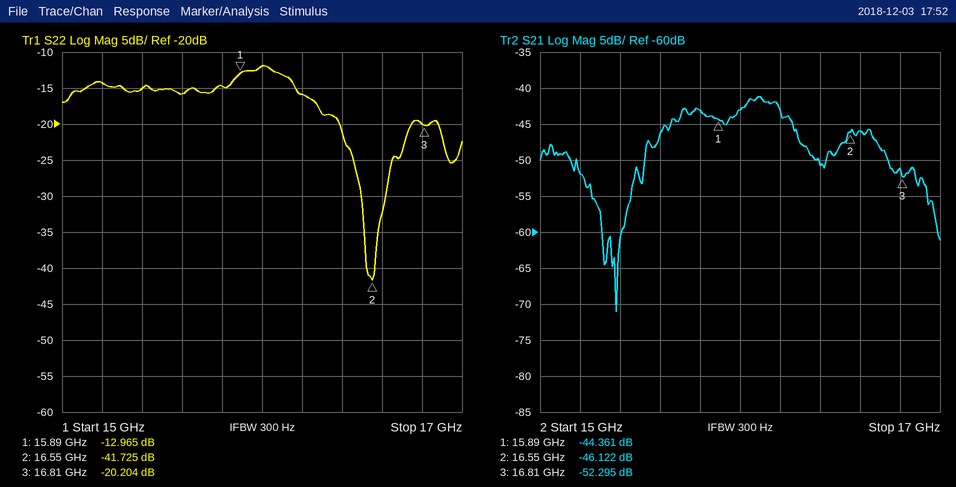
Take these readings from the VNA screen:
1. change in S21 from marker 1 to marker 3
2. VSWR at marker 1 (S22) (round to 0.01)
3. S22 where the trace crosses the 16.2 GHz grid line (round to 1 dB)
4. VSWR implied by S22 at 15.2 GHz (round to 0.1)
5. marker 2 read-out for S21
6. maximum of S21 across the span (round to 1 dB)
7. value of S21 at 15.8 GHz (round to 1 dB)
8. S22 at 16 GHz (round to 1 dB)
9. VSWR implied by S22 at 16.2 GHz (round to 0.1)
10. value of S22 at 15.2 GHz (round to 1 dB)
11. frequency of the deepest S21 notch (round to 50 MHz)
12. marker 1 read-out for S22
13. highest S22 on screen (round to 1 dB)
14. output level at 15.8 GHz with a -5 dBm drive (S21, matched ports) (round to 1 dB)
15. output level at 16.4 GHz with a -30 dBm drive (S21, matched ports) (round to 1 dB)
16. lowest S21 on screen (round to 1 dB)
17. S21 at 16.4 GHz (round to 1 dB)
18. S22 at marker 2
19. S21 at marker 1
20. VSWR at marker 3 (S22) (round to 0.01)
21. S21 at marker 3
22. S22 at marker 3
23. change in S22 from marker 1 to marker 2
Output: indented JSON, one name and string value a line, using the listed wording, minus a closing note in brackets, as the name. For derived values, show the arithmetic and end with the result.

{
  "change in S21 from marker 1 to marker 3": "-52.295 − (-44.361) = -7.934 dB",
  "VSWR at marker 1 (S22)": "(1 + 0.2248)/(1 − 0.2248) ≈ 1.58",
  "S22 where the trace crosses the 16.2 GHz grid line": "-16 dB",
  "VSWR implied by S22 at 15.2 GHz": "|Γ| = 10^(-14/20) = 0.1995; VSWR = (1 + 0.1995)/(1 − 0.1995) ≈ 1.5",
  "marker 2 read-out for S21": "-46.122 dB",
  "maximum of S21 across the span": "-41 dB",
  "value of S21 at 15.8 GHz": "-43 dB",
  "S22 at 16 GHz": "-12 dB",
  "VSWR implied by S22 at 16.2 GHz": "|Γ| = 10^(-16/20) = 0.1585; VSWR = (1 + 0.1585)/(1 − 0.1585) ≈ 1.4",
  "value of S22 at 15.2 GHz": "-14 dB",
  "frequency of the deepest S21 notch": "15.40 GHz",
  "marker 1 read-out for S22": "-12.965 dB",
  "highest S22 on screen": "-12 dB",
  "output level at 15.8 GHz with a -5 dBm drive (S21, matched ports)": "-5 dBm + (-43 dB) = -48 dBm",
  "output level at 16.4 GHz with a -30 dBm drive (S21, matched ports)": "-30 dBm + (-51 dB) = -81 dBm",
  "lowest S21 on screen": "-71 dB",
  "S21 at 16.4 GHz": "-51 dB",
  "S22 at marker 2": "-41.725 dB",
  "S21 at marker 1": "-44.361 dB",
  "VSWR at marker 3 (S22)": "(1 + 0.0977)/(1 − 0.0977) ≈ 1.22",
  "S21 at marker 3": "-52.295 dB",
  "S22 at marker 3": "-20.204 dB",
  "change in S22 from marker 1 to marker 2": "-41.725 − (-12.965) = -28.760 dB"
}
